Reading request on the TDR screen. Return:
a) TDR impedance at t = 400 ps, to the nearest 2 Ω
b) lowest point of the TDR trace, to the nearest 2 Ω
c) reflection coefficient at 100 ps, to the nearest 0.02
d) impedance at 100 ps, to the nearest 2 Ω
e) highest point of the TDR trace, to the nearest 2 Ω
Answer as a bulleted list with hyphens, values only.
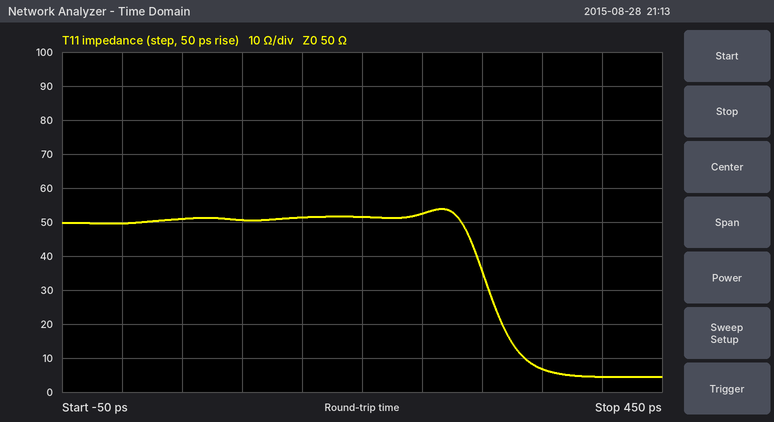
- 4 Ω
- 4 Ω
- 0.00
- 50 Ω
- 54 Ω
